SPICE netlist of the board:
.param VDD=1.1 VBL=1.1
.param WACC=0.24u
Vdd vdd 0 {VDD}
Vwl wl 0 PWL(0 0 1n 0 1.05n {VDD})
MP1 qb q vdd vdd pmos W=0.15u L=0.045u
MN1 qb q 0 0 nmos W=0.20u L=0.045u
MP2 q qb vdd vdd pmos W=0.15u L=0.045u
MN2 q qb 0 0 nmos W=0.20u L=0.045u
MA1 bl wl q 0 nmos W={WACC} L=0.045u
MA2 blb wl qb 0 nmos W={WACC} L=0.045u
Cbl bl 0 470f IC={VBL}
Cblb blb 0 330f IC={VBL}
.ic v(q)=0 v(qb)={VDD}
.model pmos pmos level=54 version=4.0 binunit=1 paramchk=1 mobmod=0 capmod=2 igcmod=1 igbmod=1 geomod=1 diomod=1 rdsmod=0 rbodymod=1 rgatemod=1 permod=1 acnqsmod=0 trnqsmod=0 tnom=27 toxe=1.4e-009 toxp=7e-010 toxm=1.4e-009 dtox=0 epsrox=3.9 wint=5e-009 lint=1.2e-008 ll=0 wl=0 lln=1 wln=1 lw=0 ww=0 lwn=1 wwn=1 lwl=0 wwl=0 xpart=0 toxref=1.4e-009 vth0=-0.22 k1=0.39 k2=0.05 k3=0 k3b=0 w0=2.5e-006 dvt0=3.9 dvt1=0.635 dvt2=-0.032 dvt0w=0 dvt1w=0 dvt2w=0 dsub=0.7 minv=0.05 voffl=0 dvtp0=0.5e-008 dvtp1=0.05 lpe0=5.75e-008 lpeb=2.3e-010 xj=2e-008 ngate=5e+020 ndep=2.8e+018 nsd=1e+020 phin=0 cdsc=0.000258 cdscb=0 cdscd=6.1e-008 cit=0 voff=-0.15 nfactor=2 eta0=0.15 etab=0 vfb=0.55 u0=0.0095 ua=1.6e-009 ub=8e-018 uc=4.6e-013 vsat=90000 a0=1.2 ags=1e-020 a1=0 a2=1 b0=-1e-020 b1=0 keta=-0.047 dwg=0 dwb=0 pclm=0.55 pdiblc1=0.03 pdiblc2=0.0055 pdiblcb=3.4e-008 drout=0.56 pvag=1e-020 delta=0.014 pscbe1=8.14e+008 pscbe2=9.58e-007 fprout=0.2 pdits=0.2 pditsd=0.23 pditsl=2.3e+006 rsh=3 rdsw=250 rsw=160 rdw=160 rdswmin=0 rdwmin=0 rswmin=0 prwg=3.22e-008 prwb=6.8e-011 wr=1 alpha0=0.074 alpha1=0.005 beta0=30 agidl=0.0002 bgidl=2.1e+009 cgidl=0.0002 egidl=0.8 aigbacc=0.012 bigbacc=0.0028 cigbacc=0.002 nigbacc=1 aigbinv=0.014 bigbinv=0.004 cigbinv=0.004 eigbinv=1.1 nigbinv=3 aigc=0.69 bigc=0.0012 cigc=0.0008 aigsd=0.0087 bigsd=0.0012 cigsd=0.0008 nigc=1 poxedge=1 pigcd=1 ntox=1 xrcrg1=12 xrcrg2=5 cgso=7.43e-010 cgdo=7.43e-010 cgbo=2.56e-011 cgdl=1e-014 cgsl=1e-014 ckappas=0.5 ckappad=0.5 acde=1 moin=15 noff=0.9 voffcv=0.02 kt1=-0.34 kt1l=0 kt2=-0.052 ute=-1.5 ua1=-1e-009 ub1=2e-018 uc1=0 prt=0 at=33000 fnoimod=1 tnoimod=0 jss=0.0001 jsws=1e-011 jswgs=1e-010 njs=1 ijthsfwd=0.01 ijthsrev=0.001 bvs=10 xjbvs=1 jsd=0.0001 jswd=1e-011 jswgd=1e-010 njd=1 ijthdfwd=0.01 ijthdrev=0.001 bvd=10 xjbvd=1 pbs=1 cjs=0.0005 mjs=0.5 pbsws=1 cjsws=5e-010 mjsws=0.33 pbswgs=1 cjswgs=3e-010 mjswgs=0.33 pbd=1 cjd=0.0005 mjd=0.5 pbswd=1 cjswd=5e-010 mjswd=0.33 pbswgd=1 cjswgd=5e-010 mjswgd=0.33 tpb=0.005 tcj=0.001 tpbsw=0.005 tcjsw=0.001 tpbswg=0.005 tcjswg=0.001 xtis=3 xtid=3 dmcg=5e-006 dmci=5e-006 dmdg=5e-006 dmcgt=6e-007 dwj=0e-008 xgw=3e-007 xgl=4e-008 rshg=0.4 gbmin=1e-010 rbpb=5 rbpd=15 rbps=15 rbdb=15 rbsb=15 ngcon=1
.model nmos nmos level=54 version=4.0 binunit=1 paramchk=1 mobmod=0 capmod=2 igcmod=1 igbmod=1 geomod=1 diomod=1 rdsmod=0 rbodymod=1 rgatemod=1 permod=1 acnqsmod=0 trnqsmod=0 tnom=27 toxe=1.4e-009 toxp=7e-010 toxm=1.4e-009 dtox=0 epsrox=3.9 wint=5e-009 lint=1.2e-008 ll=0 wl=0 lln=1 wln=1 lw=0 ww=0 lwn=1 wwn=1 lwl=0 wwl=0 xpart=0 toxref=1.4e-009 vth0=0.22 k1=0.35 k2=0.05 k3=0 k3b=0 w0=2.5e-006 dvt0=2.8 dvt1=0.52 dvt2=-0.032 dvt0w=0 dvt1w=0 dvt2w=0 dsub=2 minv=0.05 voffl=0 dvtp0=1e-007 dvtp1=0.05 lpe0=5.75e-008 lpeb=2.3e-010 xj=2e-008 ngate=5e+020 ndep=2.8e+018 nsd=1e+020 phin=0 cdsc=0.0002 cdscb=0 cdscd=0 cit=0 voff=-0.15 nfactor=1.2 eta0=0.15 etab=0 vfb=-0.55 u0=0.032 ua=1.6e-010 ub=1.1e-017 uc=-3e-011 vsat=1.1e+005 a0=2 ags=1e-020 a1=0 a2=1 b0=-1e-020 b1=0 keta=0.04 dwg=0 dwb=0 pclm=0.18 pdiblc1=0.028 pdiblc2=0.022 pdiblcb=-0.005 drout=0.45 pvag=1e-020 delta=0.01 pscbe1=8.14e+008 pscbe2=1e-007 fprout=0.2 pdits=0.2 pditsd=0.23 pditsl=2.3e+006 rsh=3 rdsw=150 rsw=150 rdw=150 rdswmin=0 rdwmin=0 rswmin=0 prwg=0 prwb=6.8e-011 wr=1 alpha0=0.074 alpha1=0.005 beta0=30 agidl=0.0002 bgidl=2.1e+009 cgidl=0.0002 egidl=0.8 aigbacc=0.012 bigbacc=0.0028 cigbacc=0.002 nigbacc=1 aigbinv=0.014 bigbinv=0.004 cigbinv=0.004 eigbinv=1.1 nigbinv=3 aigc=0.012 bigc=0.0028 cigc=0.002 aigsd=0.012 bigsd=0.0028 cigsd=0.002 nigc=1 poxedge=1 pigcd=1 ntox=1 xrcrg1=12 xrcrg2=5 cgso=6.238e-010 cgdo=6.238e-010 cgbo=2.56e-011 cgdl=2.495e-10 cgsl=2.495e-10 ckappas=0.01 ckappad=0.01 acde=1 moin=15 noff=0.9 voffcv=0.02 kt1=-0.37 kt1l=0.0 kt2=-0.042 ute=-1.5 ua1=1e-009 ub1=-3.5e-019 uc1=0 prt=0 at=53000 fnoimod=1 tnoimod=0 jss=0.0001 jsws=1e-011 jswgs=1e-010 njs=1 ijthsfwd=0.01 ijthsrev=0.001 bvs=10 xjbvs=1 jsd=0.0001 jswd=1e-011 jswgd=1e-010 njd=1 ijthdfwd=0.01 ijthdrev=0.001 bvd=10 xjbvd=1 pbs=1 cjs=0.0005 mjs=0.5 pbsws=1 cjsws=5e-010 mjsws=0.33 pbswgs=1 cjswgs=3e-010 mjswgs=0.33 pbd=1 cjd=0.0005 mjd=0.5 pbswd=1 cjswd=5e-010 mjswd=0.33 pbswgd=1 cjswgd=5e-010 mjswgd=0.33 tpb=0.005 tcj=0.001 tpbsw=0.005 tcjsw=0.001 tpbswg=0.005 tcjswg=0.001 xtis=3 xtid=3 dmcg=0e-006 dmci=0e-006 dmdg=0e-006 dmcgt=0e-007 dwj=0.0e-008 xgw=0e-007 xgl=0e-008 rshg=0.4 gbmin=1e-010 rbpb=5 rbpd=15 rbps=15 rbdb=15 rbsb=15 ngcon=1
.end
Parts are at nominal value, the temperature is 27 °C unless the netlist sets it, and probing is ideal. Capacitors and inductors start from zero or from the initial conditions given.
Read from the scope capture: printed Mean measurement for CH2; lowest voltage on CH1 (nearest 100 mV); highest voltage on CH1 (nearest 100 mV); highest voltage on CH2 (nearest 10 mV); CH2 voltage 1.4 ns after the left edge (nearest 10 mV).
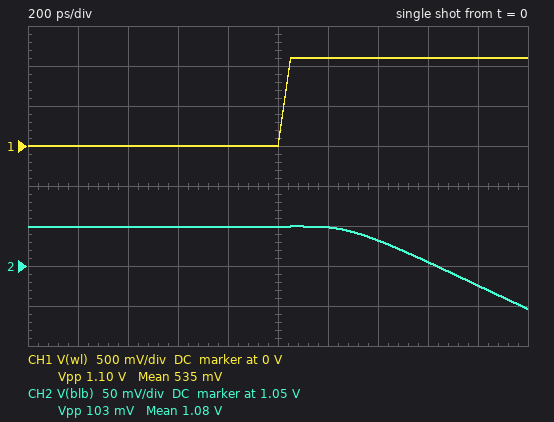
1.08 V
0 V
1.1 V
1.10 V
1.08 V
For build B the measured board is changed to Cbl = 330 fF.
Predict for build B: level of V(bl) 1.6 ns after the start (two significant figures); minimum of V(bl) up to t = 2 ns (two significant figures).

930 mV
830 mV
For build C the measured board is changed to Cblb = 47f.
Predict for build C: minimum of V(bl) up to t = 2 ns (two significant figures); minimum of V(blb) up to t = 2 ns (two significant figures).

980 mV
160 mV
